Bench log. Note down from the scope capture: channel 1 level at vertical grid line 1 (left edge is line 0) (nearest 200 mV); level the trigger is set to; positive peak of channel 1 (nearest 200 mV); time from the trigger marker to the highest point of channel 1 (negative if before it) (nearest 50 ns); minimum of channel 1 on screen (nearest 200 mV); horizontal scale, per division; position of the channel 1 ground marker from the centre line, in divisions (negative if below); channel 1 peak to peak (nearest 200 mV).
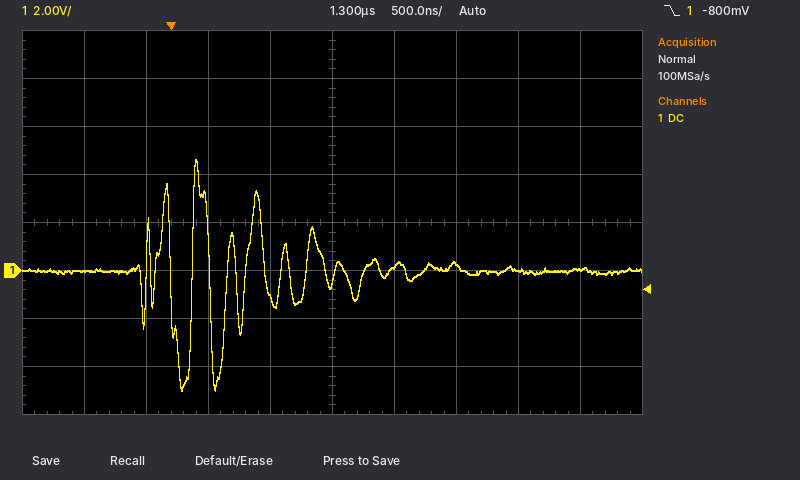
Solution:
0.0 V
-800 mV
4.6 V
+200 ns
-5.0 V
500 ns
-1.0 div
9.6 V
